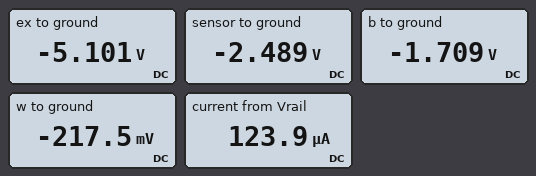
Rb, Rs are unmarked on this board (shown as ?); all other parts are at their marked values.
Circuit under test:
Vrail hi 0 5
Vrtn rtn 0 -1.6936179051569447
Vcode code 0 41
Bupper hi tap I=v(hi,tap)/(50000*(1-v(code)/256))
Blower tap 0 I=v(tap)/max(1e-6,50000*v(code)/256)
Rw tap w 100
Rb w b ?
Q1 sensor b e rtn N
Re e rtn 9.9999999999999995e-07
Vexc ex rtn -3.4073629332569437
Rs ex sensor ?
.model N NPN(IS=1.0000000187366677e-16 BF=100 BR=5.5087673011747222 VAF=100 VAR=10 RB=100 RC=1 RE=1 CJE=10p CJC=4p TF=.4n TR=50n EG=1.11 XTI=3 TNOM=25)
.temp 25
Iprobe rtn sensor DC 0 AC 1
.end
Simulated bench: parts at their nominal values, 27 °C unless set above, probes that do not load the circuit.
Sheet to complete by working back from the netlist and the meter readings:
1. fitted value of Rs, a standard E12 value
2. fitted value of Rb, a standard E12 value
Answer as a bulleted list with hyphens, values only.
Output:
- 2.7 kΩ
- 10 kΩ
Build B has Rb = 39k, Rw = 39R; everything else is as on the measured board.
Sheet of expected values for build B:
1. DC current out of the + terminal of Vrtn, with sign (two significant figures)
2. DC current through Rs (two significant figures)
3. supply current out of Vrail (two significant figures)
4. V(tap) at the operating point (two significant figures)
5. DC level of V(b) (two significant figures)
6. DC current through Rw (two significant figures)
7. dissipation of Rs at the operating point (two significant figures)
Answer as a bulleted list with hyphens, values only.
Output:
- -79 µA
- 560 µA
- 110 µA
- 270 mV
- -2.8 V
- 79 µA
- 850 µW
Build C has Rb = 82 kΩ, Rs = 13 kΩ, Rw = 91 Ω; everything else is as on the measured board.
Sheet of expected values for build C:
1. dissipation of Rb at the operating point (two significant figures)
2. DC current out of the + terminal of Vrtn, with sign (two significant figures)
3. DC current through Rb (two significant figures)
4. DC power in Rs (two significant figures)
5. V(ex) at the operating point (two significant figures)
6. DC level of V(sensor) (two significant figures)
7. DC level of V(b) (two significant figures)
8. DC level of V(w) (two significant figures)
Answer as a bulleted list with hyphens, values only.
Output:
- 73 µW
- -30 µA
- 30 µA
- 490 µW
- -5.1 V
- -2.6 V
- -1.8 V
- 600 mV
